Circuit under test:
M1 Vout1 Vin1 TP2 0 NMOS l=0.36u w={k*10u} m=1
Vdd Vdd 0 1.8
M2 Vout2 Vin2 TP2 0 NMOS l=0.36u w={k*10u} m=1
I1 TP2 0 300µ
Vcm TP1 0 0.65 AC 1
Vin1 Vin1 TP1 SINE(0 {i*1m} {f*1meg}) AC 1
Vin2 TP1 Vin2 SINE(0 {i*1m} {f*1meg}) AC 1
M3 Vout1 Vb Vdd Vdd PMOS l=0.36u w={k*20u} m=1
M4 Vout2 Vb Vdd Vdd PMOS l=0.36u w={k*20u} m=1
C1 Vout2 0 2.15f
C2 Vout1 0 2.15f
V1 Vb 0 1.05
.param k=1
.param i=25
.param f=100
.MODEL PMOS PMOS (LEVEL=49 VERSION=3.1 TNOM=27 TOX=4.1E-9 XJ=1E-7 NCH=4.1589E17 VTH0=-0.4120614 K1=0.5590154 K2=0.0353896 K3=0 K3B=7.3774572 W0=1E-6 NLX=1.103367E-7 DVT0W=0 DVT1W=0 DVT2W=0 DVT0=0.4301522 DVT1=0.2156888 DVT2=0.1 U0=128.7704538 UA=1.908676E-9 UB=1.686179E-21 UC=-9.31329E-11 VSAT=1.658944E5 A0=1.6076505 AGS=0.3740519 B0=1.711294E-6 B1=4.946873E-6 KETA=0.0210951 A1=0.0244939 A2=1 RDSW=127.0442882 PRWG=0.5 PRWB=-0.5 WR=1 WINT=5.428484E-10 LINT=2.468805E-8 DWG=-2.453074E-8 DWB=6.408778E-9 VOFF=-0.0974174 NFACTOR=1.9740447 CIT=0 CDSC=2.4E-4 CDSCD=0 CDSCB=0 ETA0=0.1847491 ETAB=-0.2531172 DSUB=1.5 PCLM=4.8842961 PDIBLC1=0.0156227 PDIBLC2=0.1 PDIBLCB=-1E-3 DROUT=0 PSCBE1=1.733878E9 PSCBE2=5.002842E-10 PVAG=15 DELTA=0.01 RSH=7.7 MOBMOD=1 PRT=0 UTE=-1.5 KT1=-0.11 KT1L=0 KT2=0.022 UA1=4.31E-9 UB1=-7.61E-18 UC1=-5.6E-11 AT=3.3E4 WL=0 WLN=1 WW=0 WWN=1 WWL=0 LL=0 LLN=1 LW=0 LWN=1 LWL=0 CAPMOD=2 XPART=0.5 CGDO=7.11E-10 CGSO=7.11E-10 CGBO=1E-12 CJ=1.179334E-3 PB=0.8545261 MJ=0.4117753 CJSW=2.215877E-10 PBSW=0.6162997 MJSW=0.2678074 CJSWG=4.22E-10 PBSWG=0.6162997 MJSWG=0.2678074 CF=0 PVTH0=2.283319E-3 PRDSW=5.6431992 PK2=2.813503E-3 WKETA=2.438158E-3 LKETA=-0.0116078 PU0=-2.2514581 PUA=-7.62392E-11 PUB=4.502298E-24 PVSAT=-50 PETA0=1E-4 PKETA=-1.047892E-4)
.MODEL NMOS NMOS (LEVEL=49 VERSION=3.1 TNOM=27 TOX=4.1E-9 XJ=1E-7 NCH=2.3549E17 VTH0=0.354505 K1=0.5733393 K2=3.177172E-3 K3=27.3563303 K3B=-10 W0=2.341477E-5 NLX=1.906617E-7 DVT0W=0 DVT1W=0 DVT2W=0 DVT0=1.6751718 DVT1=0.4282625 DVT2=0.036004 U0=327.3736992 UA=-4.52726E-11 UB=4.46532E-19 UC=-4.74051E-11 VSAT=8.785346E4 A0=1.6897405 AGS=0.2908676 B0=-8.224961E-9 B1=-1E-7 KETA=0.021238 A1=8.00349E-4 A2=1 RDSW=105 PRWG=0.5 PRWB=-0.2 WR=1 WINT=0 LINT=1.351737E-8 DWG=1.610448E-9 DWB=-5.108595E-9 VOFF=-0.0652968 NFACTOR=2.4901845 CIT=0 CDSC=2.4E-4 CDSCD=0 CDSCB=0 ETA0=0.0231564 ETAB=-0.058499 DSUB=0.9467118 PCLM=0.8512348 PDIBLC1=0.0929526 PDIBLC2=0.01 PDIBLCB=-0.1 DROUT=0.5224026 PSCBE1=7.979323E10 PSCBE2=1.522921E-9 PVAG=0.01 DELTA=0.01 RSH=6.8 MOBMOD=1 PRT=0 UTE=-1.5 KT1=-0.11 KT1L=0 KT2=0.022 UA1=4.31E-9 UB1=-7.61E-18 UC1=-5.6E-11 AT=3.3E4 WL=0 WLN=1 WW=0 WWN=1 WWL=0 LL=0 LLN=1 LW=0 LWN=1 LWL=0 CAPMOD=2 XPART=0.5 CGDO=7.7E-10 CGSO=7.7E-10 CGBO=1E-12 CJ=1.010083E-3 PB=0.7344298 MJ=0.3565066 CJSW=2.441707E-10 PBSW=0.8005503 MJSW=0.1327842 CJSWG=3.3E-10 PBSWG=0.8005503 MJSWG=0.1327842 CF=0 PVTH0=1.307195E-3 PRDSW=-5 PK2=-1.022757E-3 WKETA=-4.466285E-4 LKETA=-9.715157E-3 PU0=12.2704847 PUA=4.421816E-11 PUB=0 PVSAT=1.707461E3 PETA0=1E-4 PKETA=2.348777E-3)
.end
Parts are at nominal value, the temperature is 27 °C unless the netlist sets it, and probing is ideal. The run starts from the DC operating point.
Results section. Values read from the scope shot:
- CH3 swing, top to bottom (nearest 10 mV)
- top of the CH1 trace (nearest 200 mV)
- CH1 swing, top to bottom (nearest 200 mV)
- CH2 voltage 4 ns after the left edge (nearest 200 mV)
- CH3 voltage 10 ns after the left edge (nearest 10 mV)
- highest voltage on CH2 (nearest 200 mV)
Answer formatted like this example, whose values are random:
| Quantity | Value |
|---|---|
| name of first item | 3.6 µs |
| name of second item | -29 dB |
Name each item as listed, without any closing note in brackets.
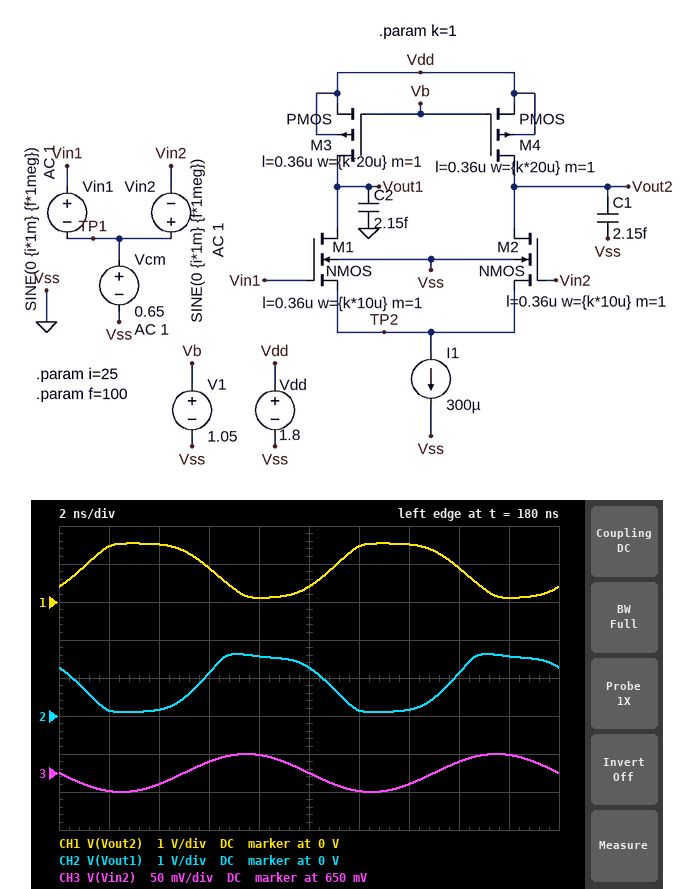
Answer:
| Quantity | Value |
|---|---|
| CH3 swing, top to bottom | 50 mV |
| top of the CH1 trace | 1.6 V |
| CH1 swing, top to bottom | 1.4 V |
| CH2 voltage 4 ns after the left edge | 200 mV |
| CH3 voltage 10 ns after the left edge | 650 mV |
| highest voltage on CH2 | 1.6 V |
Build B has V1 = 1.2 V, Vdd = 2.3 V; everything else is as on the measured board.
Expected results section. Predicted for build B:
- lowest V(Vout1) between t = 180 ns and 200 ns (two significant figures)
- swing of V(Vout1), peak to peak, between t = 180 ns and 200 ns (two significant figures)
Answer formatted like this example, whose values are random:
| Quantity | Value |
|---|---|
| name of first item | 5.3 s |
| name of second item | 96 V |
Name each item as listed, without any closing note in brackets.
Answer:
| Quantity | Value |
|---|---|
| lowest V(Vout1) between t = 180 ns and 200 ns | 2.2 V |
| swing of V(Vout1), peak to peak, between t = 180 ns and 200 ns | 36 mV |
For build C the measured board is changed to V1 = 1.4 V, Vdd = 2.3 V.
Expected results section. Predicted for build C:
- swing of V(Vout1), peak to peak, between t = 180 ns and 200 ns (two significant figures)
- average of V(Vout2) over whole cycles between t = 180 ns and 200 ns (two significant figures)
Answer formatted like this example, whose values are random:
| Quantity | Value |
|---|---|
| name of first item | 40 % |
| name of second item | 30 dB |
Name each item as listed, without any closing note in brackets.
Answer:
| Quantity | Value |
|---|---|
| swing of V(Vout1), peak to peak, between t = 180 ns and 200 ns | 62 mV |
| average of V(Vout2) over whole cycles between t = 180 ns and 200 ns | 2.2 V |
